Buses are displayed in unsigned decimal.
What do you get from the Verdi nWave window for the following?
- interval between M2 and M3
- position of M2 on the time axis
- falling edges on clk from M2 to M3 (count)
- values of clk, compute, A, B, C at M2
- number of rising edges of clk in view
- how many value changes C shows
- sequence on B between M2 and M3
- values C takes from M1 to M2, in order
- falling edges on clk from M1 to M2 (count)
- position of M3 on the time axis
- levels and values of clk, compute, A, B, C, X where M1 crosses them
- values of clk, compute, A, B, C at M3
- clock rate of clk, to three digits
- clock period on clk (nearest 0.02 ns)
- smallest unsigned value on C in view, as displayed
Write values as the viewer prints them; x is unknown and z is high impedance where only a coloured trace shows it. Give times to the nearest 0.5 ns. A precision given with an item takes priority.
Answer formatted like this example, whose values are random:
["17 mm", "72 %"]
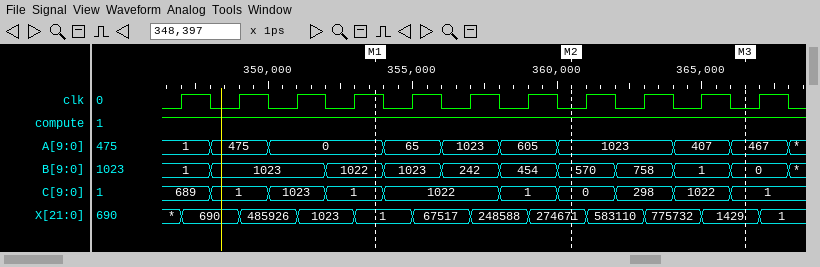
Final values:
["6 ns", "360.5 ns", "3", "clk=0, compute=1, A=1023, B=570, C=0", "11", "9", "570, 758, 1, 0", "1, 1022, 1, 0", "4", "366.5 ns", "clk=1, compute=1, A=0, B=1022, C=1, X=1", "clk=0, compute=1, A=467, B=0, C=1", "500 MHz", "2 ns", "0"]
